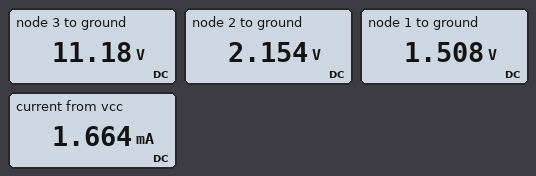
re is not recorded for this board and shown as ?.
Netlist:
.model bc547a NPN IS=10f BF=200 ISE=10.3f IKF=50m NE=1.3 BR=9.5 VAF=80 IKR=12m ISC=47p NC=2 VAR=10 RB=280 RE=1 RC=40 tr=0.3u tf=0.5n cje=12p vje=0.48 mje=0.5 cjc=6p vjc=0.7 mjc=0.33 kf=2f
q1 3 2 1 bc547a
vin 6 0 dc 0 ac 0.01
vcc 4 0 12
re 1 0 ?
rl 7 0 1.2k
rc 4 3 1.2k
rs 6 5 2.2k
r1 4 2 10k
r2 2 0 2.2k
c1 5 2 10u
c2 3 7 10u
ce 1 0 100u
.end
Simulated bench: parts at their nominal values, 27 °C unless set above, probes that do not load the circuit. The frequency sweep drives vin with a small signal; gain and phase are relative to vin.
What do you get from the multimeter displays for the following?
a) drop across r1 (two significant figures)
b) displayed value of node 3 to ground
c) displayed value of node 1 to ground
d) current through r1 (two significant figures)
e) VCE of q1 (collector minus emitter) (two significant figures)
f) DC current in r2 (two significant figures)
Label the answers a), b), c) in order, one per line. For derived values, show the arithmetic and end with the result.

a) 12 V - 2.154 V = 9.8 V
b) 11.18 V
c) 1.508 V
d) (12 V - 2.154 V) / 10 kΩ = 980 µA
e) 11.18 V - 1.508 V = 9.7 V
f) (2.154 V) / 2.2 kΩ = 980 µA
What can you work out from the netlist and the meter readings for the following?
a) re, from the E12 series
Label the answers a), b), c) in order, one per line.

a) 2.2 kΩ
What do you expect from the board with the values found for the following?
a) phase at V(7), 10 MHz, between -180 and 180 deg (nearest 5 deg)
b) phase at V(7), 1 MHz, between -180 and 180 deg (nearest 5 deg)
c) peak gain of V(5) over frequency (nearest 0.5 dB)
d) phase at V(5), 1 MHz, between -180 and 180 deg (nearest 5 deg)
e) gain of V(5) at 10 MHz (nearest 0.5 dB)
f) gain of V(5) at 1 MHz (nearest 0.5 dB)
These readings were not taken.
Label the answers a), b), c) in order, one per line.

a) 95 deg
b) 150 deg
c) 0 dB
d) -20 deg
e) -18.5 dB
f) -9.5 dB
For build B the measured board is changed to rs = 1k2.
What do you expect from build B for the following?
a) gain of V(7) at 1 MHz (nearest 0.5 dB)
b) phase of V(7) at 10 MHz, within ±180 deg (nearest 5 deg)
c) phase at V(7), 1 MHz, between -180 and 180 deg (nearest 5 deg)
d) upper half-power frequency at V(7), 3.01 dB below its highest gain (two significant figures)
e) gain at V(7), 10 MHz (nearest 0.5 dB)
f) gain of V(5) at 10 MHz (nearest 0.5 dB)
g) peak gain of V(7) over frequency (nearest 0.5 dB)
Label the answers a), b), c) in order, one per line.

a) 17.0 dB
b) 100 deg
c) 155 deg
d) 2.2 MHz
e) 4.0 dB
f) -14.0 dB
g) 17.5 dB
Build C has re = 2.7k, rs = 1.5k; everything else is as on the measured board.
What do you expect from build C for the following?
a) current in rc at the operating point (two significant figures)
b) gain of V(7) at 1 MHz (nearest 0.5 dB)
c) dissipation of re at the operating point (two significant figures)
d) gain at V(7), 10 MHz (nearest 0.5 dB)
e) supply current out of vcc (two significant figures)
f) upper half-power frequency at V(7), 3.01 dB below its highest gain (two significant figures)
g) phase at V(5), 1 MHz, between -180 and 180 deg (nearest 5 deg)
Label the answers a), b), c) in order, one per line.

a) 560 µA
b) 14.5 dB
c) 850 µW
d) 2.0 dB
e) 1.5 mA
f) 2.2 MHz
g) -15 deg
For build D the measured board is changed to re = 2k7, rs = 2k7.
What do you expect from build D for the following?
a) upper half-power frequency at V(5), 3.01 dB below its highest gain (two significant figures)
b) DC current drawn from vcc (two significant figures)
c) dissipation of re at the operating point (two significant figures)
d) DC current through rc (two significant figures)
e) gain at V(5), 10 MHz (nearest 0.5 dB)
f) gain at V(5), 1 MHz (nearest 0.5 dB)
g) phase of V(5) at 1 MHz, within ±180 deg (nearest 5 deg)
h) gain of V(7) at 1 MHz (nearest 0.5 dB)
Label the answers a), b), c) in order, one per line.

a) 4.4 Hz
b) 1.5 mA
c) 850 µW
d) 560 µA
e) -19.5 dB
f) -10.5 dB
g) -20 deg
h) 11.0 dB
